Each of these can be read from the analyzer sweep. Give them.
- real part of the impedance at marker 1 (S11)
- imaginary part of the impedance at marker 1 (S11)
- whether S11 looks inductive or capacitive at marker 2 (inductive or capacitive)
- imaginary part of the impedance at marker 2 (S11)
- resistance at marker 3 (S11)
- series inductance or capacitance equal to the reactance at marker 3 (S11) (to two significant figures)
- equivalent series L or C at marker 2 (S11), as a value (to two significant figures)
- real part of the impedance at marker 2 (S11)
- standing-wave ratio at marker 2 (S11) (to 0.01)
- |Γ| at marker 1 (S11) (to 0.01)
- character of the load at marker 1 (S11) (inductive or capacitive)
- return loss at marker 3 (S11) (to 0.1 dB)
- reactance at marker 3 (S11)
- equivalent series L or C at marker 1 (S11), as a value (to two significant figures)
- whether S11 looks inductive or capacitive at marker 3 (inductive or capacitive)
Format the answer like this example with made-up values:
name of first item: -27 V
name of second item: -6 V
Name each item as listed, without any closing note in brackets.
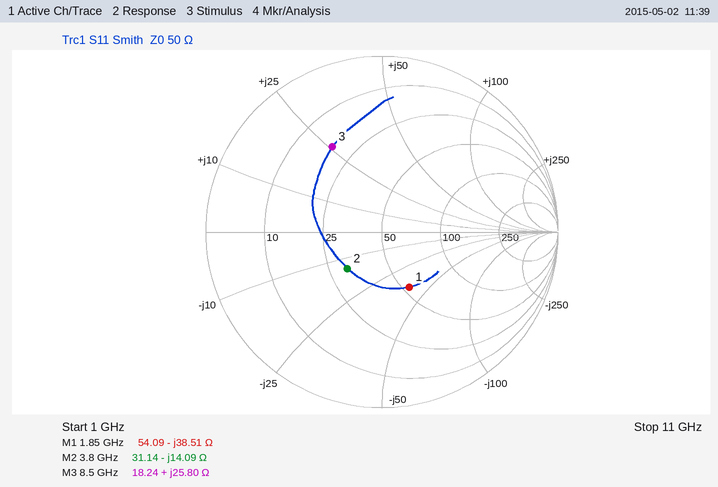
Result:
real part of the impedance at marker 1: 54.09 Ω
imaginary part of the impedance at marker 1: -38.51 Ω
whether S11 looks inductive or capacitive at marker 2: capacitive
imaginary part of the impedance at marker 2: -14.09 Ω
resistance at marker 3: 18.24 Ω
series inductance or capacitance equal to the reactance at marker 3 (S11): 480 pH
equivalent series L or C at marker 2 (S11), as a value: 3.0 pF
real part of the impedance at marker 2: 31.14 Ω
standing-wave ratio at marker 2 (S11): 1.80
|Γ| at marker 1 (S11): 0.35
character of the load at marker 1 (S11): capacitive
return loss at marker 3 (S11): 5.0 dB
reactance at marker 3: +25.80 Ω
equivalent series L or C at marker 1 (S11), as a value: 2.2 pF
whether S11 looks inductive or capacitive at marker 3: inductive
